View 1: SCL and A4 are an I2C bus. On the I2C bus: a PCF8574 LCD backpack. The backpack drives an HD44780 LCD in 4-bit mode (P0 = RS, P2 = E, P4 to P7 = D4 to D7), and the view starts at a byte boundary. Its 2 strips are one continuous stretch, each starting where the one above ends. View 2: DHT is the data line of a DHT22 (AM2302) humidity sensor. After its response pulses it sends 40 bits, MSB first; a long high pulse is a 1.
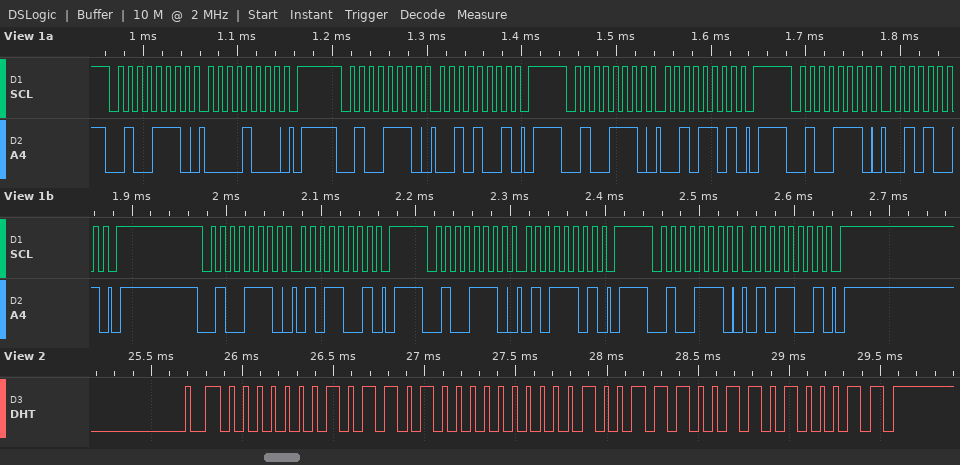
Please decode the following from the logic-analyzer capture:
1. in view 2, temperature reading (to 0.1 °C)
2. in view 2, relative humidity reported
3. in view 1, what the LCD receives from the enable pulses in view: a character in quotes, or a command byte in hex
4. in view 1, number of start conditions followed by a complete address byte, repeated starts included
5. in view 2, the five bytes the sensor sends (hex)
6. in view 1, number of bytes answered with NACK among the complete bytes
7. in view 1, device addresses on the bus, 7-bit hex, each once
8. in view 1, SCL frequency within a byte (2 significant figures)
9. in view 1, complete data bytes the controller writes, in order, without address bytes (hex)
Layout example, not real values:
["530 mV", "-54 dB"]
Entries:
["31.3 °C", "36.0 %", "'%'", "7", "01 68 01 39 A3", "0", "0x27", "100 kHz", "08 29 2D 29 59 5D 59"]
